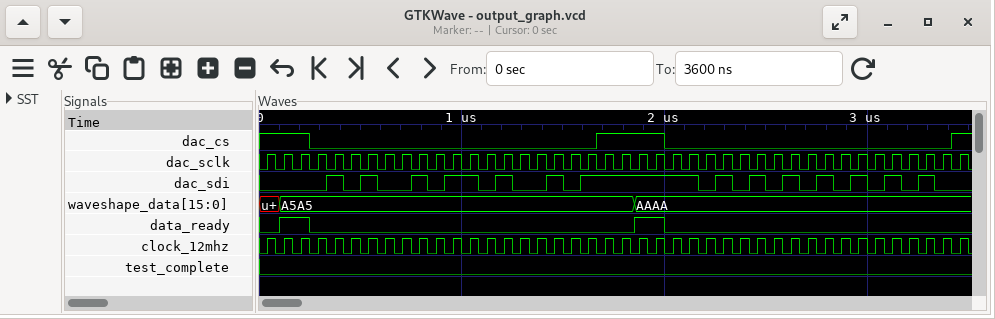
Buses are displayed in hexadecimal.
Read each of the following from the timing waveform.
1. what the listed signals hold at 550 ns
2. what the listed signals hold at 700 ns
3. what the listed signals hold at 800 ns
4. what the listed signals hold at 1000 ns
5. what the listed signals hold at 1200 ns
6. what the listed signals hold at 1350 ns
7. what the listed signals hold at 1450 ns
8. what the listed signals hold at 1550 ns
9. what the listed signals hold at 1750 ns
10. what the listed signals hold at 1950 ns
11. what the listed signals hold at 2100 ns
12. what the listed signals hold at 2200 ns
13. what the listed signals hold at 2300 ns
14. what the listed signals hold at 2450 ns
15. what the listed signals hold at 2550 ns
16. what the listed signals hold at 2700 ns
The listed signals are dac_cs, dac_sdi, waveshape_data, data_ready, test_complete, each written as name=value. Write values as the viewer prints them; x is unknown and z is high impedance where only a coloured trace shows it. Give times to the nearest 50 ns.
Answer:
dac_cs=0, dac_sdi=1, waveshape_data=A5A5, data_ready=0, test_complete=0
dac_cs=0, dac_sdi=0, waveshape_data=A5A5, data_ready=0, test_complete=0
dac_cs=0, dac_sdi=1, waveshape_data=A5A5, data_ready=0, test_complete=0
dac_cs=0, dac_sdi=1, waveshape_data=A5A5, data_ready=0, test_complete=0
dac_cs=0, dac_sdi=1, waveshape_data=A5A5, data_ready=0, test_complete=0
dac_cs=0, dac_sdi=0, waveshape_data=A5A5, data_ready=0, test_complete=0
dac_cs=0, dac_sdi=1, waveshape_data=A5A5, data_ready=0, test_complete=0
dac_cs=0, dac_sdi=0, waveshape_data=A5A5, data_ready=0, test_complete=0
dac_cs=1, dac_sdi=1, waveshape_data=A5A5, data_ready=0, test_complete=0
dac_cs=1, dac_sdi=1, waveshape_data=AAAA, data_ready=1, test_complete=0
dac_cs=0, dac_sdi=1, waveshape_data=AAAA, data_ready=0, test_complete=0
dac_cs=0, dac_sdi=0, waveshape_data=AAAA, data_ready=0, test_complete=0
dac_cs=0, dac_sdi=1, waveshape_data=AAAA, data_ready=0, test_complete=0
dac_cs=0, dac_sdi=1, waveshape_data=AAAA, data_ready=0, test_complete=0
dac_cs=0, dac_sdi=0, waveshape_data=AAAA, data_ready=0, test_complete=0
dac_cs=0, dac_sdi=0, waveshape_data=AAAA, data_ready=0, test_complete=0
